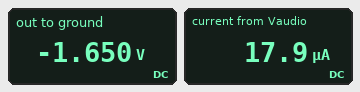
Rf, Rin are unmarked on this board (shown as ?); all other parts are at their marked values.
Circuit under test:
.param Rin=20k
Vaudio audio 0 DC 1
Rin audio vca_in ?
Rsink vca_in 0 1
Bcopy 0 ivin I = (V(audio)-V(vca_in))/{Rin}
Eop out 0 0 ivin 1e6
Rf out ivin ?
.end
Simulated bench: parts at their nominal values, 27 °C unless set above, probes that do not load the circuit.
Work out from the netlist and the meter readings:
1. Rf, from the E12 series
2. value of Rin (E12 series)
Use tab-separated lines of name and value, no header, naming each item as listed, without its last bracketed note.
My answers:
Rf, from the E12 series	33 kΩ
value of Rin	56 kΩ
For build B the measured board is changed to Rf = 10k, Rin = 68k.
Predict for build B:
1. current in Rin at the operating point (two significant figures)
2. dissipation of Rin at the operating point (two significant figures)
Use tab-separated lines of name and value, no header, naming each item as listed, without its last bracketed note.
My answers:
current in Rin at the operating point	15 µA
dissipation of Rin at the operating point	15 µW
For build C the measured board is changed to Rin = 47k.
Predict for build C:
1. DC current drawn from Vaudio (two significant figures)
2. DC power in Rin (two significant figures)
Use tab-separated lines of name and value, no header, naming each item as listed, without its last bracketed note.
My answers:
DC current drawn from Vaudio	21 µA
DC power in Rin	21 µW
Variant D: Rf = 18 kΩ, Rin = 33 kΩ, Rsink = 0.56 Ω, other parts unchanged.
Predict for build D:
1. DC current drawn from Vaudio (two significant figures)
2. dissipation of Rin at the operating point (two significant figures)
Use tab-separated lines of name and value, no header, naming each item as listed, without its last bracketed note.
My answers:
DC current drawn from Vaudio	30 µA
dissipation of Rin at the operating point	30 µW
